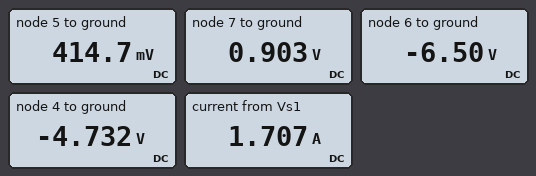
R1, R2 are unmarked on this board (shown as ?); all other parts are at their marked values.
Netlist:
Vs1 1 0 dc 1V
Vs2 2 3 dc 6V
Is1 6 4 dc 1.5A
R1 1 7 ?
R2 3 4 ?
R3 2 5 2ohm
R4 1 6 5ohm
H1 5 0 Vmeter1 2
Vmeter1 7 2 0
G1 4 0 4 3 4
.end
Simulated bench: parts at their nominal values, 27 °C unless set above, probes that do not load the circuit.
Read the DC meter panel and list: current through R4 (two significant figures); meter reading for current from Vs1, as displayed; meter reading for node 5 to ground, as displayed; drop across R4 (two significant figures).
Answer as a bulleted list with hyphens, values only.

- 1.5 A
- 1.707 A
- 414.7 mV
- 7.5 V
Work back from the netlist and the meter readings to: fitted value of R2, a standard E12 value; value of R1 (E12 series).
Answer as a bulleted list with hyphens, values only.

- 10 Ω
- 0.47 Ω
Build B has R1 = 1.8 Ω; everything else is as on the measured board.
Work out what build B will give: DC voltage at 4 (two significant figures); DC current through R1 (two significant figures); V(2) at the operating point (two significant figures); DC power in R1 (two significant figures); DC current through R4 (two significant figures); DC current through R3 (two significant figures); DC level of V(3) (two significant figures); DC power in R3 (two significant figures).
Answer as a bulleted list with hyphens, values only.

- -4.9 V
- 160 mA
- 710 mV
- 46 mW
- 1.5 A
- 200 mA
- -5.3 V
- 77 mW
